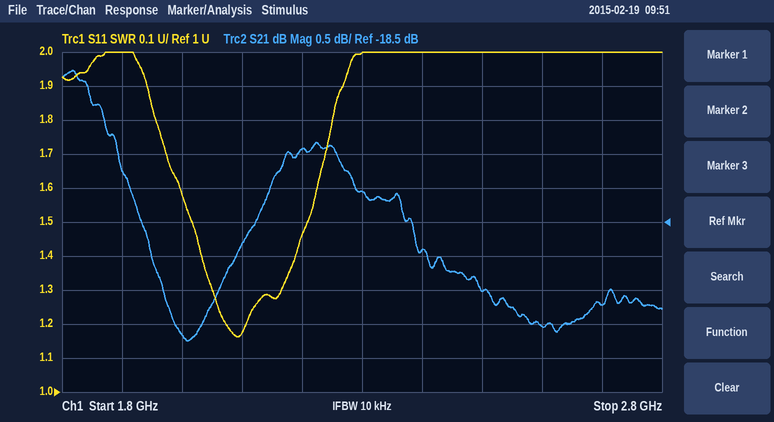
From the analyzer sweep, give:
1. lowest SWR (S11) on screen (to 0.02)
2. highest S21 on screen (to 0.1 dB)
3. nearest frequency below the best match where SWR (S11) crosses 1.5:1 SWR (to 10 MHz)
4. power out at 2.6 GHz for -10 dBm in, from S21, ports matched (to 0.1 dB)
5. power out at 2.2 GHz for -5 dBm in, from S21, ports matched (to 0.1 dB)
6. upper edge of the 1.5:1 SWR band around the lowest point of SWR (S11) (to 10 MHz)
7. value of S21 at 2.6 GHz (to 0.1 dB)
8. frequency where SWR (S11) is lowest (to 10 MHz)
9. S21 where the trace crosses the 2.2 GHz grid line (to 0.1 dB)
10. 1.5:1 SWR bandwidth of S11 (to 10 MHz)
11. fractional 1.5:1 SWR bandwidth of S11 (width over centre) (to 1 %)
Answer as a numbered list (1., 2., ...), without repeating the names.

1. 1.16
2. -16.3 dB
3. 2.02 GHz
4. -30.0 dBm
5. -22.4 dBm
6. 2.21 GHz
7. -20.0 dB
8. 2.09 GHz
9. -17.4 dB
10. 190 MHz
11. 9 %
